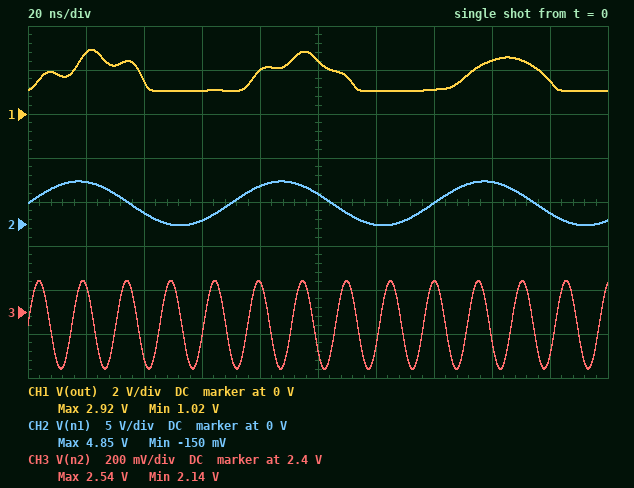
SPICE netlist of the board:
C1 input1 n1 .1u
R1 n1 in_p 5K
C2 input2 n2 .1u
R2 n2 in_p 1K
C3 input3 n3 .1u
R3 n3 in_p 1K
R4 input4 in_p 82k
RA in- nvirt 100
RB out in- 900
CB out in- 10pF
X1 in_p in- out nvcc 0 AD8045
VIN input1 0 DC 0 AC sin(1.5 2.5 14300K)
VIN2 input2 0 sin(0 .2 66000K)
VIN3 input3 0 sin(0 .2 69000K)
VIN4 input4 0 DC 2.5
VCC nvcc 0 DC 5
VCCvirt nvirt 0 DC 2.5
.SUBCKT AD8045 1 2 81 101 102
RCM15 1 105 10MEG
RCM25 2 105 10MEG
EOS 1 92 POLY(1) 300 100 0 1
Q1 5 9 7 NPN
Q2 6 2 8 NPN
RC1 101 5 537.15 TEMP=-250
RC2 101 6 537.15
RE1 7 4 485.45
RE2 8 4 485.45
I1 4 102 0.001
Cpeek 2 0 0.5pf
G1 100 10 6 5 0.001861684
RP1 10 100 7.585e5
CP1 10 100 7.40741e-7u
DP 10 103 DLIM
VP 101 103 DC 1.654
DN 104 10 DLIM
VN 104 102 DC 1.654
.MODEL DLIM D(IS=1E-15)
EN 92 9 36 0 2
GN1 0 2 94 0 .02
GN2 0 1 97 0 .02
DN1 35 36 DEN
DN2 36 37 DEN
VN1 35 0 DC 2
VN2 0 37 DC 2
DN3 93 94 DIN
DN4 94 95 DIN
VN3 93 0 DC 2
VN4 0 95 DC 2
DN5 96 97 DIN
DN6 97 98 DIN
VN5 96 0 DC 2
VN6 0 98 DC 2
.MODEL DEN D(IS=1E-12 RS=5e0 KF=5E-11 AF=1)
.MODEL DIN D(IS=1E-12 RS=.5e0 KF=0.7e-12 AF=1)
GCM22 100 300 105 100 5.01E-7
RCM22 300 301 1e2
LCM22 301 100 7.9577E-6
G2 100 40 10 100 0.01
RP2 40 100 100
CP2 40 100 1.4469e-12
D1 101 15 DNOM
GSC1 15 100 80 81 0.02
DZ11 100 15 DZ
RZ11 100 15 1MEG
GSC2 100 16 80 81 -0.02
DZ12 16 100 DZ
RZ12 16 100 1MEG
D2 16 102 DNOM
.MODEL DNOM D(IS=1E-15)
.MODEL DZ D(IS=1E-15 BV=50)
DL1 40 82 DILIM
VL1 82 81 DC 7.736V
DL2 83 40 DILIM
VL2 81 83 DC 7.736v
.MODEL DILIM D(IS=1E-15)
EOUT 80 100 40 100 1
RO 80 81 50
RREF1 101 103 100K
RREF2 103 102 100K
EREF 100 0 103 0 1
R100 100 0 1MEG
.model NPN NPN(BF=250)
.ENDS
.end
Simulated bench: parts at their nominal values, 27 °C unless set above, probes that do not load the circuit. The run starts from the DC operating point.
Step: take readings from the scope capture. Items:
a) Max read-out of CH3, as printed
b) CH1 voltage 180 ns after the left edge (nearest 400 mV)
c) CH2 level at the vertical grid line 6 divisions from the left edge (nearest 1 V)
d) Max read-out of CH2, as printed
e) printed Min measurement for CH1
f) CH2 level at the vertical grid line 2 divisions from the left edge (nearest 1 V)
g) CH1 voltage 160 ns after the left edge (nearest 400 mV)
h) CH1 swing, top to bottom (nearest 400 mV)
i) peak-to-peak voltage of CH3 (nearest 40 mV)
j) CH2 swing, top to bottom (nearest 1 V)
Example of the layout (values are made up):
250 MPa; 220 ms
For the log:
2.54 V; 1.6 V; 0 V; 4.85 V; 1.02 V; 1 V; 2.4 V; 2.0 V; 400 mV; 5 V
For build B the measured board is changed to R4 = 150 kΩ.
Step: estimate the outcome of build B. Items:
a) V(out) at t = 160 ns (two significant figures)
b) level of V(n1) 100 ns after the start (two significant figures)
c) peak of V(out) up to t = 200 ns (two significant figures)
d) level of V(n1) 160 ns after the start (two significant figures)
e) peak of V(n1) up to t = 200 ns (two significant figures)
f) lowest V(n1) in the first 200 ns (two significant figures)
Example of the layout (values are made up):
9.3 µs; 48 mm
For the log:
1.8 V; 3.3 V; 2.2 V; 4.7 V; 4.8 V; -240 mV
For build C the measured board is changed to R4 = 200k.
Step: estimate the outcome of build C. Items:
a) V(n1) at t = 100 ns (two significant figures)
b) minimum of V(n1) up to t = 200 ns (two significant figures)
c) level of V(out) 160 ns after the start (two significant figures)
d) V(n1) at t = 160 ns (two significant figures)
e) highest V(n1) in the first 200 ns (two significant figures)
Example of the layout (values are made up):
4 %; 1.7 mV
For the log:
3.3 V; -290 mV; 1.5 V; 4.6 V; 4.7 V
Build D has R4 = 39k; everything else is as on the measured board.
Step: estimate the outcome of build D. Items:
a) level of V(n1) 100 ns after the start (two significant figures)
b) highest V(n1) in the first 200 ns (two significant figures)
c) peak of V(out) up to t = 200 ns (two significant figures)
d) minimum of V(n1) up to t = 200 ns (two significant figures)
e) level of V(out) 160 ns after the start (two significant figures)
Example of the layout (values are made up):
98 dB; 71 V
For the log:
3.5 V; 4.9 V; 3.7 V; -78 mV; 3.1 V
